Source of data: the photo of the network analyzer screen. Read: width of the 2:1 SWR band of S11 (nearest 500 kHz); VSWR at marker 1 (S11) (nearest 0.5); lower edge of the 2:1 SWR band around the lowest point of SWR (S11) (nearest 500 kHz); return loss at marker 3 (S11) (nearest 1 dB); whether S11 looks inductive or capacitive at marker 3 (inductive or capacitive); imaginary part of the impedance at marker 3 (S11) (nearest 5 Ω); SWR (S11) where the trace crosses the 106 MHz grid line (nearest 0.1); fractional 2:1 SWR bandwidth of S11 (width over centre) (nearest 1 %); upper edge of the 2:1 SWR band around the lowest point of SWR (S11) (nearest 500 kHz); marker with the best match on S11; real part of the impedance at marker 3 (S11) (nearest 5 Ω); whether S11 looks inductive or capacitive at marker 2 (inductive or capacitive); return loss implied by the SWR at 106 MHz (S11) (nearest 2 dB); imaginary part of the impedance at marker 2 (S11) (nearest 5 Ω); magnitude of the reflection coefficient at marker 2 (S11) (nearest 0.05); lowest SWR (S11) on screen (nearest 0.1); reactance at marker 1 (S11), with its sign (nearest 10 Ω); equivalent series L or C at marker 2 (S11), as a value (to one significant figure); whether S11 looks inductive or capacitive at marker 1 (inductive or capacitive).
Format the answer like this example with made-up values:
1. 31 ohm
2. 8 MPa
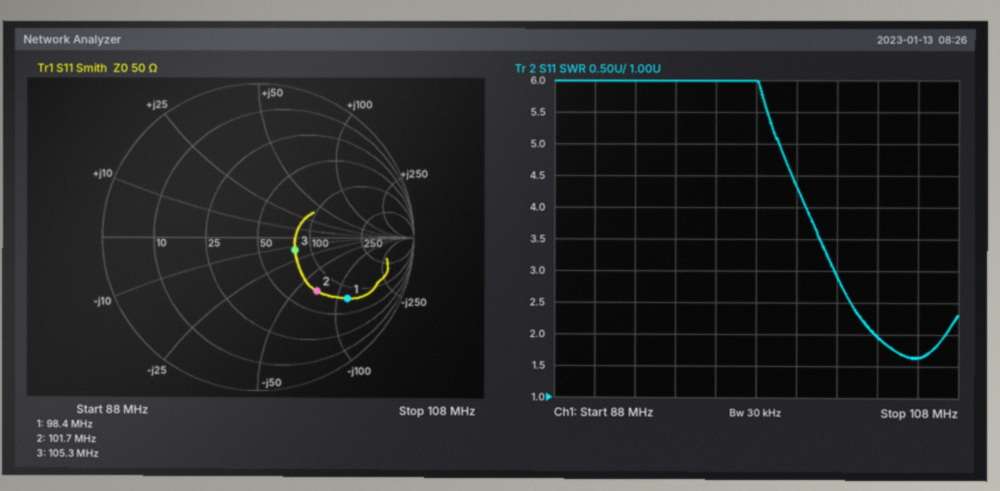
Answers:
1. 3.5 MHz
2. 5.5
3. 104.0 MHz
4. 12 dB
5. capacitive
6. -15 Ω
7. 1.6
8. 3 %
9. 107.5 MHz
10. marker 3
11. 80 Ω
12. capacitive
13. 12 dB
14. -70 Ω
15. 0.50
16. 1.6
17. -120 Ω
18. 20 pF
19. capacitive
